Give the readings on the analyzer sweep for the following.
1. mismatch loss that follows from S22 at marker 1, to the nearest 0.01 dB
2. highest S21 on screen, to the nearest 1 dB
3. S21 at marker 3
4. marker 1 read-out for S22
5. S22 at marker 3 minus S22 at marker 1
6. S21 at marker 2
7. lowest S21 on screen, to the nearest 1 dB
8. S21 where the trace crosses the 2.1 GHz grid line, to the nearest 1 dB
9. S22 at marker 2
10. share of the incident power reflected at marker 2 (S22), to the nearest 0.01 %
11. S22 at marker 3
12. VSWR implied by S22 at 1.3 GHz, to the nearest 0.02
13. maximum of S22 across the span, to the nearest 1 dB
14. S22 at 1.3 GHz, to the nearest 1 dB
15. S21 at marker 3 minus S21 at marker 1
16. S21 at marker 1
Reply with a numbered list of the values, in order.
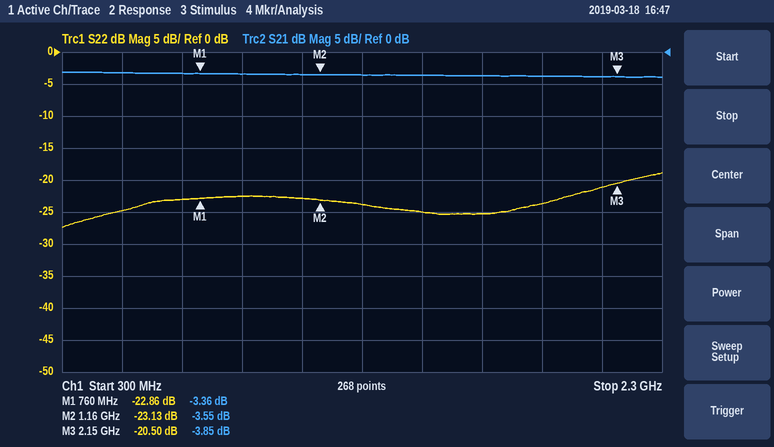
1. 0.02 dB
2. -3 dB
3. -3.85 dB
4. -22.86 dB
5. 2.36 dB
6. -3.55 dB
7. -4 dB
8. -4 dB
9. -23.13 dB
10. 0.49 %
11. -20.50 dB
12. 1.14
13. -19 dB
14. -24 dB
15. -0.49 dB
16. -3.36 dB
